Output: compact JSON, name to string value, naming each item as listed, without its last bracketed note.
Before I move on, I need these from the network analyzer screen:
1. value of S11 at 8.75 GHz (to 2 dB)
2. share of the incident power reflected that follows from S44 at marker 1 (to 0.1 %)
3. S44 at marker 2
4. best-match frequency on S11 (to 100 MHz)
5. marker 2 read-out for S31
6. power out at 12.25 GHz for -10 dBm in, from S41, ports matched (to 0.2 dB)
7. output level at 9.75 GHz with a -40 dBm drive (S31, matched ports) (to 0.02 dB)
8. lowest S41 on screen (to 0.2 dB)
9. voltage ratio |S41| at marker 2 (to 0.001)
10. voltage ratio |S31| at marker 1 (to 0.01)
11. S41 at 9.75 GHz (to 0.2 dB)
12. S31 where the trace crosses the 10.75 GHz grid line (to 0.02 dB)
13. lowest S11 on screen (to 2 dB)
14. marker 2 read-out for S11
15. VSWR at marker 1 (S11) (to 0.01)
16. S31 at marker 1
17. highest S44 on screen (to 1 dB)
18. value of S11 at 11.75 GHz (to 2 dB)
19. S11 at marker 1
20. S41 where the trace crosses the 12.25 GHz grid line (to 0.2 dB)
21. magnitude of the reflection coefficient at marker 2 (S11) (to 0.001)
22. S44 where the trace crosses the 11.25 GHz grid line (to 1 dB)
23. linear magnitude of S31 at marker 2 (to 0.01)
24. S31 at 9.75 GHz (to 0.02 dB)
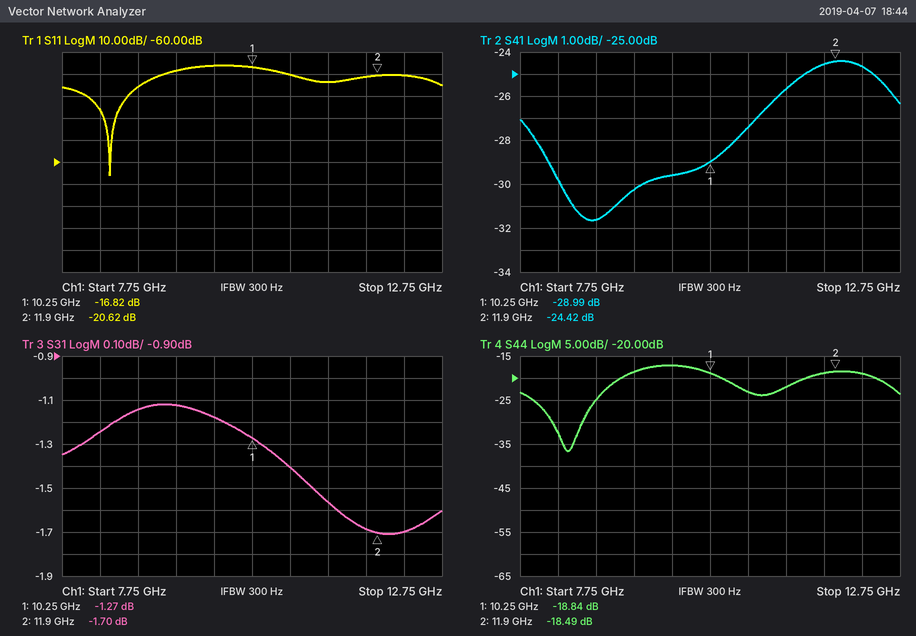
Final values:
{"value of S11 at 8.75 GHz": "-26 dB", "share of the incident power reflected that follows from S44 at marker 1": "1.3 %", "S44 at marker 2": "-18.49 dB", "best-match frequency on S11": "8.4 GHz", "marker 2 read-out for S31": "-1.70 dB", "power out at 12.25 GHz for -10 dBm in, from S41, ports matched": "-34.6 dBm", "output level at 9.75 GHz with a -40 dBm drive (S31, matched ports)": "-41.18 dBm", "lowest S41 on screen": "-31.6 dB", "voltage ratio |S41| at marker 2": "0.060", "voltage ratio |S31| at marker 1": "0.86", "S41 at 9.75 GHz": "-29.6 dB", "S31 where the trace crosses the 10.75 GHz grid line": "-1.40 dB", "lowest S11 on screen": "-66 dB", "marker 2 read-out for S11": "-20.62 dB", "VSWR at marker 1 (S11)": "1.34", "S31 at marker 1": "-1.27 dB", "highest S44 on screen": "-17 dB", "value of S11 at 11.75 GHz": "-22 dB", "S11 at marker 1": "-16.82 dB", "S41 where the trace crosses the 12.25 GHz grid line": "-24.6 dB", "magnitude of the reflection coefficient at marker 2 (S11)": "0.093", "S44 where the trace crosses the 11.25 GHz grid line": "-22 dB", "linear magnitude of S31 at marker 2": "0.82", "S31 at 9.75 GHz": "-1.18 dB"}
